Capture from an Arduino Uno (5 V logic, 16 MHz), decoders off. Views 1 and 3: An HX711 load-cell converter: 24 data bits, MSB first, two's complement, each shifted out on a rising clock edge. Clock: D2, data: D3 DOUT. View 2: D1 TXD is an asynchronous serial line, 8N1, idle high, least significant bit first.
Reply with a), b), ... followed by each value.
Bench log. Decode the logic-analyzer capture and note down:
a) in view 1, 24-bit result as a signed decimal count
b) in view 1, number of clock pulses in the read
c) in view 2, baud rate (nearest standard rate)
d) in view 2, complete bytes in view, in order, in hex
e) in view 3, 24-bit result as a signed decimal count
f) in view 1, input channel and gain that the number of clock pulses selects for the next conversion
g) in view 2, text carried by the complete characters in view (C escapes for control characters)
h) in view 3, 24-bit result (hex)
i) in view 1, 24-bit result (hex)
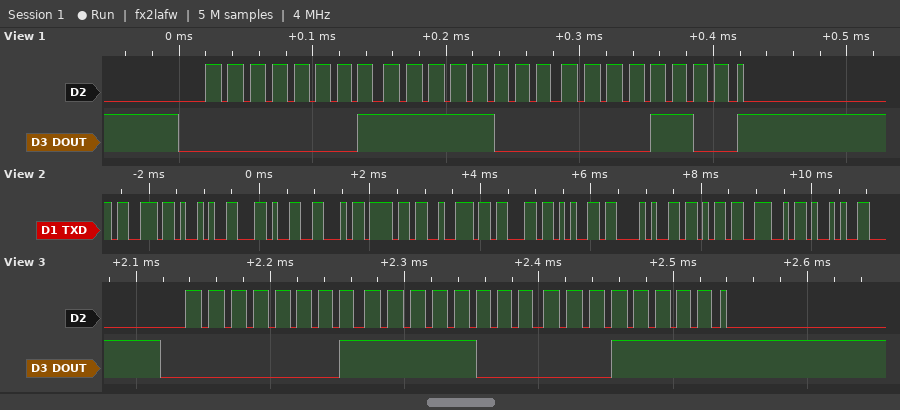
a) 129036
b) 25
c) 9600 baud
d) 0x73 0x29 0x2C 0x46 0x6F 0x72 0x63 0x65 0x28 0x6B 0x4E 0x29
e) 129055
f) channel A, gain 128
g) "s),Force(kN)"
h) 0x01F81F
i) 0x01F80C
